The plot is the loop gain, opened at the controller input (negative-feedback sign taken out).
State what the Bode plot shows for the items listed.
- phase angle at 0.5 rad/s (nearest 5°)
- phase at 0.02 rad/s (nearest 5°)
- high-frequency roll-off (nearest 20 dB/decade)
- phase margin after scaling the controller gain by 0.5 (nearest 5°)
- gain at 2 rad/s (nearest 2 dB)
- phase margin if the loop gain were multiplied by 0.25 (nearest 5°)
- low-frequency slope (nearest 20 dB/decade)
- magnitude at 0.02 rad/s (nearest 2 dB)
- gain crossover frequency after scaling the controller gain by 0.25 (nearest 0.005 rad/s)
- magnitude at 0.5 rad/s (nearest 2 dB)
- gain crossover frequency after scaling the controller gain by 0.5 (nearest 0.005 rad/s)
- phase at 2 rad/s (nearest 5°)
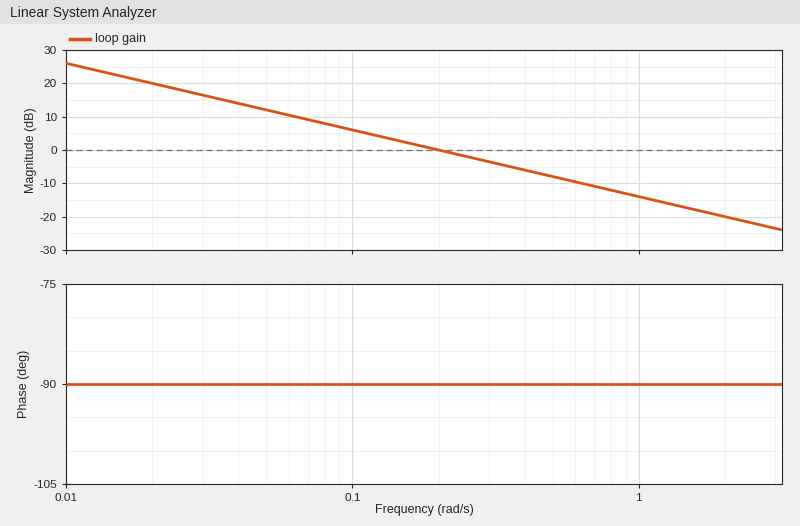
-90°
-90°
-20 dB/decade
90°
-20 dB
90°
-20 dB/decade
20 dB
0.050 rad/s
-8 dB
0.100 rad/s
-90°
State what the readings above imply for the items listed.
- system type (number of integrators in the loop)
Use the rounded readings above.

1
